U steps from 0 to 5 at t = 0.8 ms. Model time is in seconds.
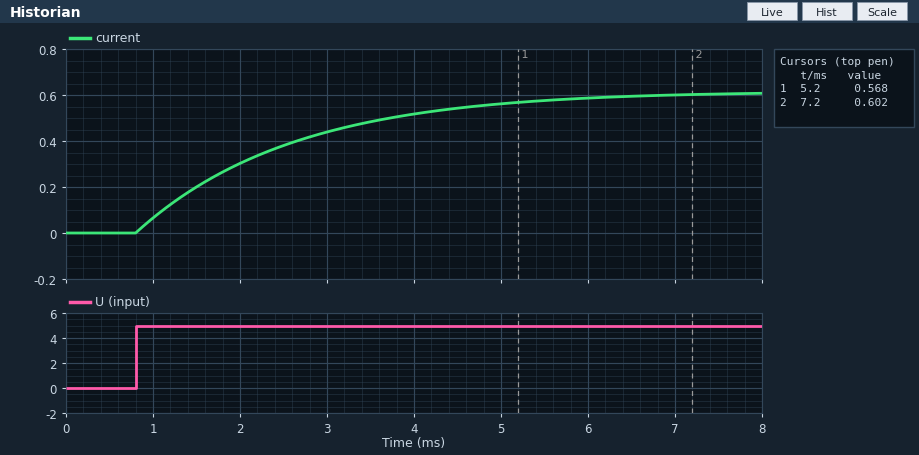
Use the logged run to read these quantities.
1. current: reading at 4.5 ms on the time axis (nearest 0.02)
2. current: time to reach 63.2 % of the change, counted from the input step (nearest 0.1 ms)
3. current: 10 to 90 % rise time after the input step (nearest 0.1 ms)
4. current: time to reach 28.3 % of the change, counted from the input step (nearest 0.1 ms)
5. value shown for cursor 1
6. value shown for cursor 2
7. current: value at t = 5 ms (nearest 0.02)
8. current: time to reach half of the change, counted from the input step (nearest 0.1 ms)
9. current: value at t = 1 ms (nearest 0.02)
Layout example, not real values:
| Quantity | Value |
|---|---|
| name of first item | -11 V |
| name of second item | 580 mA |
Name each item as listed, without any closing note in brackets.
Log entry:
| Quantity | Value |
|---|---|
| current: reading at 4.5 ms on the time axis | 0.54 |
| current: time to reach 63.2 % of the change, counted from the input step | 1.7 ms |
| current: 10 to 90 % rise time after the input step | 3.6 ms |
| current: time to reach 28.3 % of the change, counted from the input step | 0.6 ms |
| value shown for cursor 1 | 0.568 |
| value shown for cursor 2 | 0.602 |
| current: value at t = 5 ms | 0.56 |
| current: time to reach half of the change, counted from the input step | 1.2 ms |
| current: value at t = 1 ms | 0.06 |
